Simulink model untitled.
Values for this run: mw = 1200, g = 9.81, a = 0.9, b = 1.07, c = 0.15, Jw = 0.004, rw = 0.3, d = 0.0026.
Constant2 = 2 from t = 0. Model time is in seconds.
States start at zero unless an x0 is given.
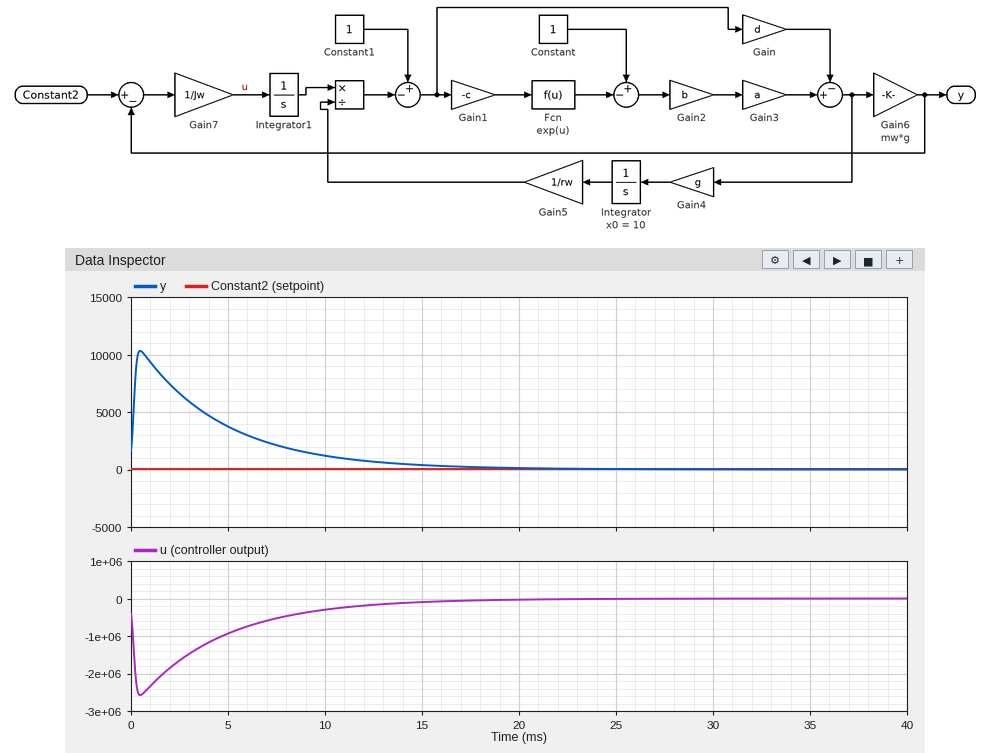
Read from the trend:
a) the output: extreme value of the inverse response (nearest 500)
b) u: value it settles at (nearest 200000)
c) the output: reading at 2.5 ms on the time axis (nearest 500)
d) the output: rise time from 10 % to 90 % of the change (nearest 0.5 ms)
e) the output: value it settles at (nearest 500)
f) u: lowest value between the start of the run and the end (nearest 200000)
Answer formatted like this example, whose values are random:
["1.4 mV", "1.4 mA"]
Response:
["10500", "0", "6500", "9.5 ms", "0", "-2600000"]
